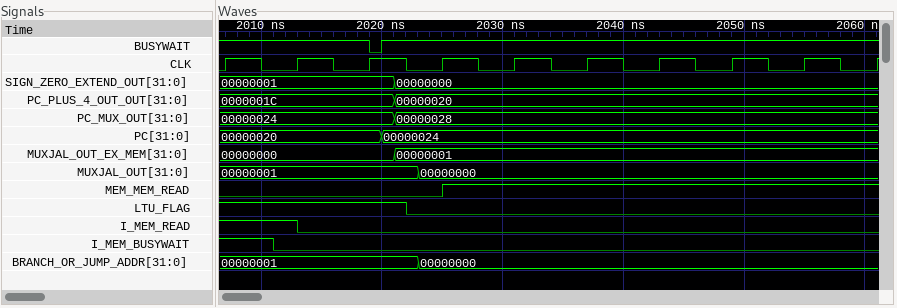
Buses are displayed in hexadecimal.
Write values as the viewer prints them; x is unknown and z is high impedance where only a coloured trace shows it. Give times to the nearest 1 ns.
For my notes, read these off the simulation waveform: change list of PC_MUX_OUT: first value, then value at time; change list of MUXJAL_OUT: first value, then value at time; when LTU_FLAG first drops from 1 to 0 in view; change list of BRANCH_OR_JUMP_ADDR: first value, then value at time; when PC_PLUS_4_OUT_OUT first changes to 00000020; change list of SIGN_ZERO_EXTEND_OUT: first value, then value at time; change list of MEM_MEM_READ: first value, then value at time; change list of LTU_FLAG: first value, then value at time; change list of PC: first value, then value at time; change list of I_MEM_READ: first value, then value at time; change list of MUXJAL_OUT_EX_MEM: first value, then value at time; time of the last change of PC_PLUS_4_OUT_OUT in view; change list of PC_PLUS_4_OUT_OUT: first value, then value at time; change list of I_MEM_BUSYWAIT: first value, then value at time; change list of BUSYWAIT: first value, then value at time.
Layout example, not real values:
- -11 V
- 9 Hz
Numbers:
- 00000024, 00000028 at 2021 ns
- 00000001, 00000000 at 2023 ns
- 2022 ns
- 00000001, 00000000 at 2023 ns
- 2021 ns
- 00000001, 00000000 at 2021 ns
- 0, 1 at 2025 ns
- 1, 0 at 2022 ns
- 00000020, 00000024 at 2020 ns
- 1, 0 at 2013 ns
- 00000000, 00000001 at 2021 ns
- 2021 ns
- 0000001C, 00000020 at 2021 ns
- 1, 0 at 2011 ns
- 1, 0 at 2019 ns, 1 at 2020 ns
